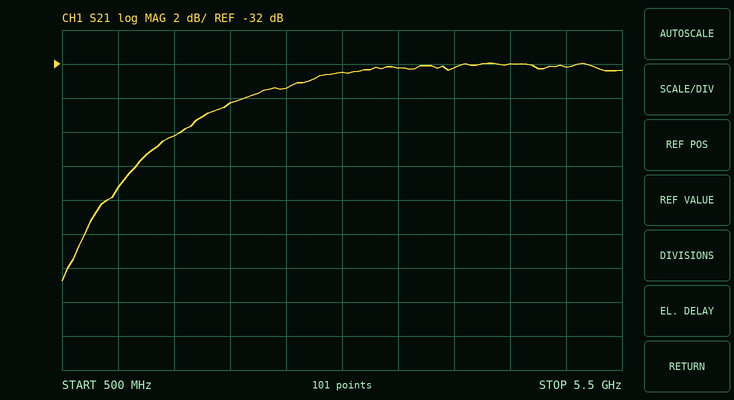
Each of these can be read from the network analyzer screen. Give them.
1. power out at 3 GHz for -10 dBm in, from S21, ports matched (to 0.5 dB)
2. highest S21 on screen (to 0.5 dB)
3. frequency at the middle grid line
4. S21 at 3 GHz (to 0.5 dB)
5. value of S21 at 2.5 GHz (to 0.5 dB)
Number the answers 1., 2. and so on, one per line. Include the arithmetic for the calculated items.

1. -10 dBm + (-32.5 dB) = -42.5 dBm
2. -32.0 dB
3. 3 GHz
4. -32.5 dB
5. -33.5 dB
